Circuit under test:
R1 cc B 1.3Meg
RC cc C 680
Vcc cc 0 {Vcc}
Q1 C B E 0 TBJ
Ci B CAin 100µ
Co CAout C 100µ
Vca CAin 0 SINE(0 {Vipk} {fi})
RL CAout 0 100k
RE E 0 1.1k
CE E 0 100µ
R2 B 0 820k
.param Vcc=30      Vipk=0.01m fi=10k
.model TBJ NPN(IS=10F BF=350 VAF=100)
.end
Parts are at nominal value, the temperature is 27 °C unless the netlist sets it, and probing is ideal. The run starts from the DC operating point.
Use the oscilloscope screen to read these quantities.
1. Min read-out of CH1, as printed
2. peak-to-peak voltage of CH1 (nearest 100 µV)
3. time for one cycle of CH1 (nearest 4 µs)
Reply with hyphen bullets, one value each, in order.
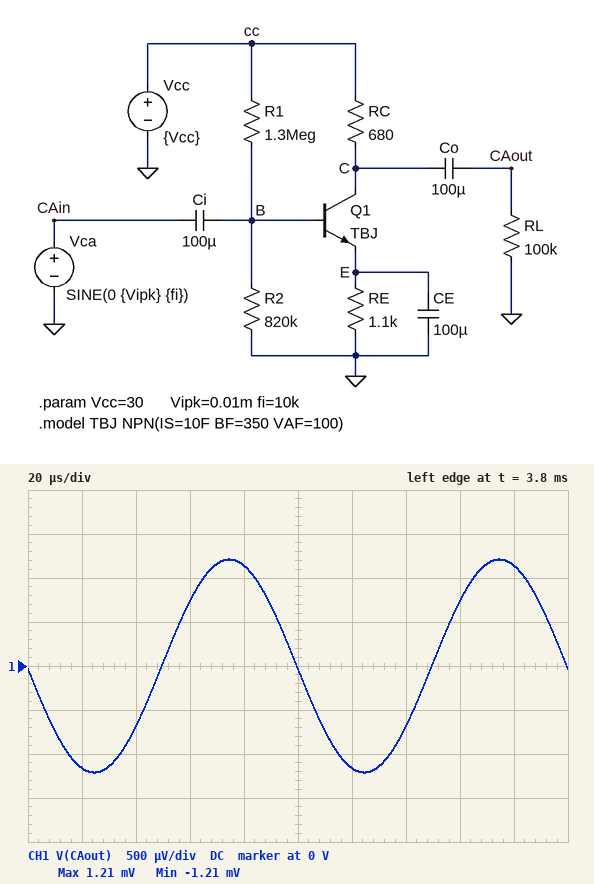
- -1.21 mV
- 2.4 mV
- 100 µs
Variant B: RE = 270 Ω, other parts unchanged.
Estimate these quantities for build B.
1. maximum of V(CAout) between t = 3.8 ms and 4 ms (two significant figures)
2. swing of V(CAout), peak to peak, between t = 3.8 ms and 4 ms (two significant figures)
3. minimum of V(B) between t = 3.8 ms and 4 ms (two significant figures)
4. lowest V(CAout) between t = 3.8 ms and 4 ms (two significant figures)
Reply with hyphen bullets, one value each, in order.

- 1.9 mV
- 3.8 mV
- 2.7 V
- -1.9 mV
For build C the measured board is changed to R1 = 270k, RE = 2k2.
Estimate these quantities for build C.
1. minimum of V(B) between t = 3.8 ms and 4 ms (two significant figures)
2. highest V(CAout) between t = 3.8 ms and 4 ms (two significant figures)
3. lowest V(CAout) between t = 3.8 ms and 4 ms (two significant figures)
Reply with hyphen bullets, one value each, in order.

- 18 V
- 2.0 mV
- -2.0 mV
